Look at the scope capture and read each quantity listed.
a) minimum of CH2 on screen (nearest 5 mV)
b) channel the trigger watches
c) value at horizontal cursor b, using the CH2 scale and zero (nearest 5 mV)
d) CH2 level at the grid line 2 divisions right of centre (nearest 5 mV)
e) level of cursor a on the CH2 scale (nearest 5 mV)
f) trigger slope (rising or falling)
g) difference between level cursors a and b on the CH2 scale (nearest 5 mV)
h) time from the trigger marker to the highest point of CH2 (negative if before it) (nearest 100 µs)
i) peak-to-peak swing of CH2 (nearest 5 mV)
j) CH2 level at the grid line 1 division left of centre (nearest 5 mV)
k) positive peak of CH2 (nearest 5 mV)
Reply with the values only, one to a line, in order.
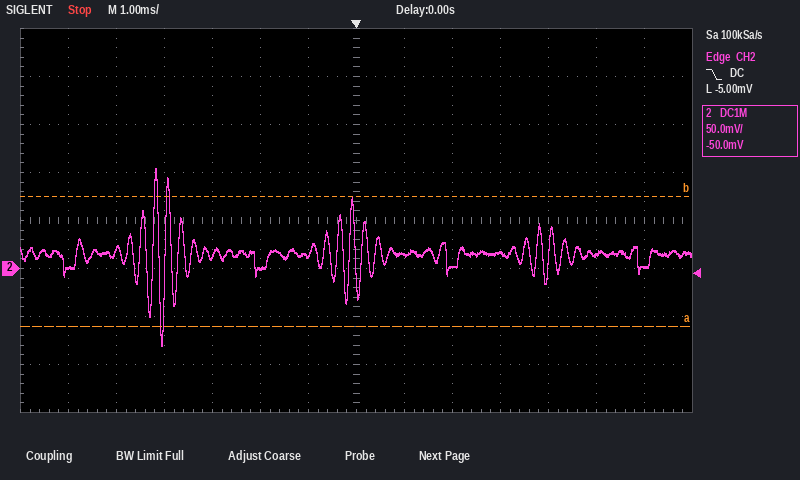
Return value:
-80 mV
CH2
75 mV
0 mV
-60 mV
falling
135 mV
-4.2 ms
185 mV
15 mV
105 mV
